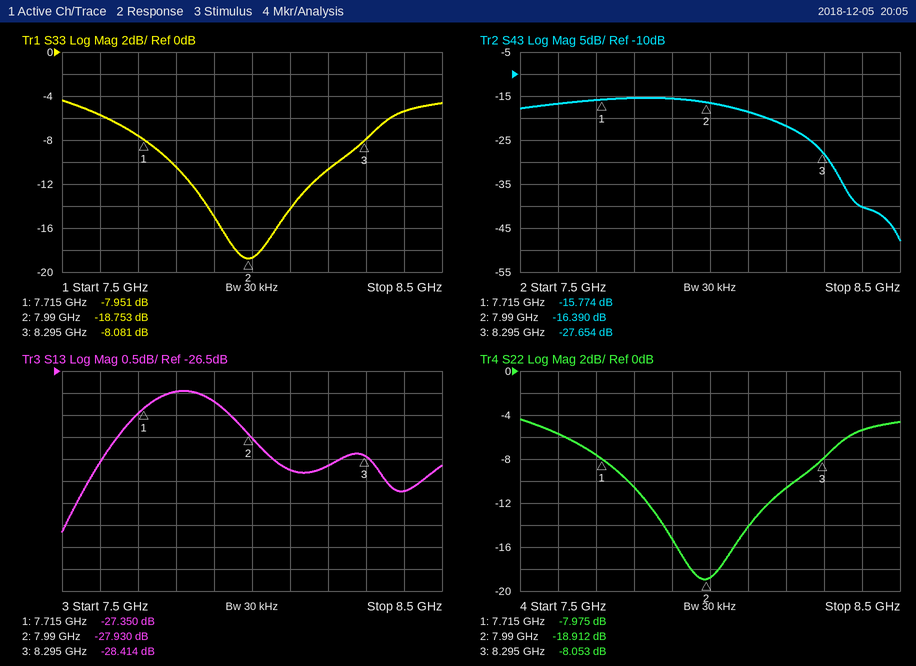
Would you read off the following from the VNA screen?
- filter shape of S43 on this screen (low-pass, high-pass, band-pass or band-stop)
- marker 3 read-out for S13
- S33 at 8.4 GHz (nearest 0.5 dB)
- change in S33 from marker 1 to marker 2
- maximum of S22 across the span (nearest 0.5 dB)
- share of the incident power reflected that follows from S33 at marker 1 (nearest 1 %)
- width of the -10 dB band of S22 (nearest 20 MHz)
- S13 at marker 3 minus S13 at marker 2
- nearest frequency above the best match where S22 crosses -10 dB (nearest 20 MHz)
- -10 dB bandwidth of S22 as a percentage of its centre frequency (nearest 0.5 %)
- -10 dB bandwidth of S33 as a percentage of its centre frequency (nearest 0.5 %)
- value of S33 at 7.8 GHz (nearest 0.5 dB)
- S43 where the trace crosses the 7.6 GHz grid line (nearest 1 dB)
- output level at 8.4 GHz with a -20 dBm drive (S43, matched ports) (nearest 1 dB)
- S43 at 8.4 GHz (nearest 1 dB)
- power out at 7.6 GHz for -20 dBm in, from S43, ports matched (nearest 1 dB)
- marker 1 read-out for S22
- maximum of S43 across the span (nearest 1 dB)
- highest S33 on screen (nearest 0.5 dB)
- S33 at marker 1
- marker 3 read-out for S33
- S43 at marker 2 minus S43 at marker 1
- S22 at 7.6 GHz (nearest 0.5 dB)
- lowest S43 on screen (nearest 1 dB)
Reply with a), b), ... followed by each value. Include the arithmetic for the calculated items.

a) low-pass
b) -28.414 dB
c) -5.5 dB
d) -18.753 − (-7.951) = -10.802 dB
e) -4.5 dB
f) 10^(-7.951/10) ≈ 16 %
g) 8.22 GHz − 7.78 GHz = 440 MHz
h) -28.414 − (-27.93) = -0.484 dB
i) 8.22 GHz
j) 440 MHz / 8 GHz ≈ 5.5 %
k) 440 MHz / 8 GHz ≈ 5.5 %
l) -10.5 dB
m) -17 dB
n) -20 dBm + (-40 dB) = -60 dBm
o) -40 dB
p) -20 dBm + (-17 dB) = -37 dBm
q) -7.975 dB
r) -15 dB
s) -4.5 dB
t) -7.951 dB
u) -8.081 dB
v) -16.39 − (-15.774) = -0.616 dB
w) -5.5 dB
x) -48 dB
